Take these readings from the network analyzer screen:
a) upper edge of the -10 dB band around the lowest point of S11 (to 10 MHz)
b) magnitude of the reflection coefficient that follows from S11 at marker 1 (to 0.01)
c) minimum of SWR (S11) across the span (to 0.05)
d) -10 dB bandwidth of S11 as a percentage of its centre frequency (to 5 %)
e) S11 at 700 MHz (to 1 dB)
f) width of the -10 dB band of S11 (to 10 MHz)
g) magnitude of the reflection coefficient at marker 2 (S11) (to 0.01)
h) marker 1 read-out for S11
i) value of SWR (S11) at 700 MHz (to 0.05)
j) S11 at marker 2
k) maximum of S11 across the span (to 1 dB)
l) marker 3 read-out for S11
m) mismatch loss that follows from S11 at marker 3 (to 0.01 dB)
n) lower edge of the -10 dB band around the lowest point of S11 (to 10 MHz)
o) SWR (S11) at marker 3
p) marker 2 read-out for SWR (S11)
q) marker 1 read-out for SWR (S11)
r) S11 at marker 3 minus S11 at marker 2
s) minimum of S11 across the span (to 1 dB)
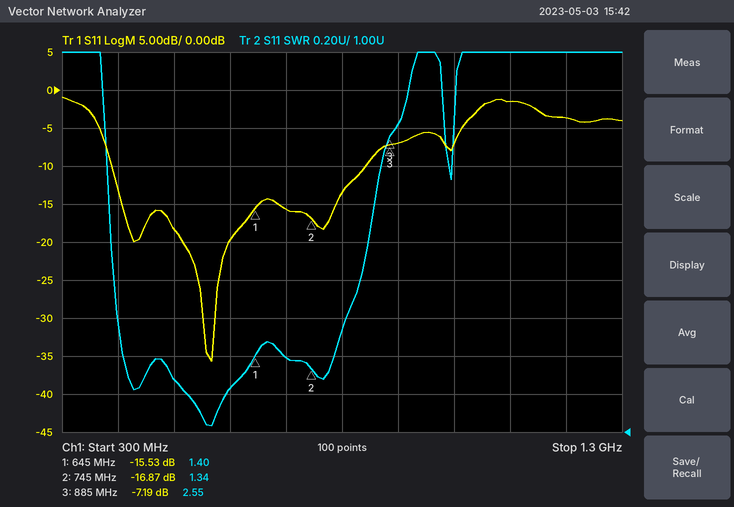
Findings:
840 MHz
0.17
1.05
75 %
-16 dB
450 MHz
0.14
-15.53 dB
1.40
-16.87 dB
-1 dB
-7.19 dB
0.92 dB
390 MHz
2.55
1.34
1.40
9.68 dB
-36 dB
